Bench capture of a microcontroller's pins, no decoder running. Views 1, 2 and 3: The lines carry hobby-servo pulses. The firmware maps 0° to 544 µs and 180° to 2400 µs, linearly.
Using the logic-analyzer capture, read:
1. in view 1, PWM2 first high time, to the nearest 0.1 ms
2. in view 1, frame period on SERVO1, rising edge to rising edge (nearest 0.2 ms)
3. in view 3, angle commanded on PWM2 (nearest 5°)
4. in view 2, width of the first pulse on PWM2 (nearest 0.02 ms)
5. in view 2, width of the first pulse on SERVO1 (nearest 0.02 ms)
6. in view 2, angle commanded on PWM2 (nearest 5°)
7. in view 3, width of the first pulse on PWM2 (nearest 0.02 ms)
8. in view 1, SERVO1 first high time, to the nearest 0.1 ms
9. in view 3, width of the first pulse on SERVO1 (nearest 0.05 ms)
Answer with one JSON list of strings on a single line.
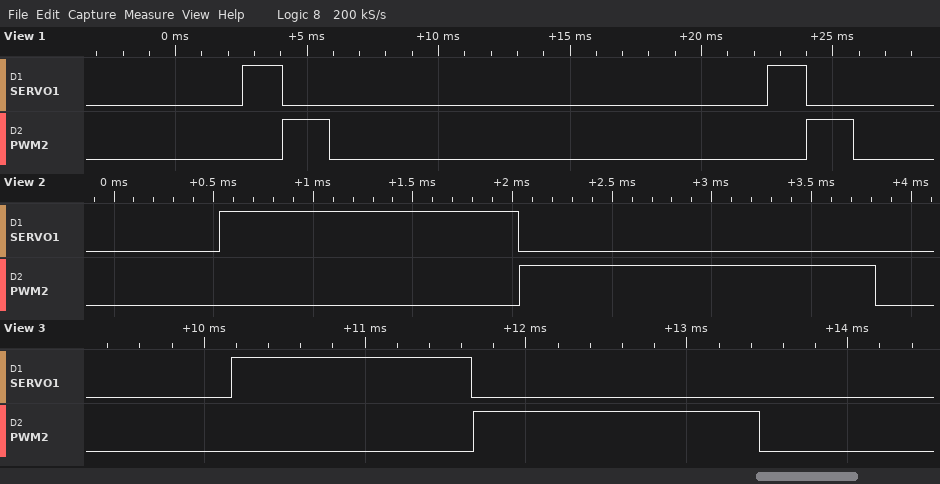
["1.8 ms", "20.0 ms", "120°", "1.78 ms", "1.50 ms", "120°", "1.78 ms", "1.5 ms", "1.50 ms"]
